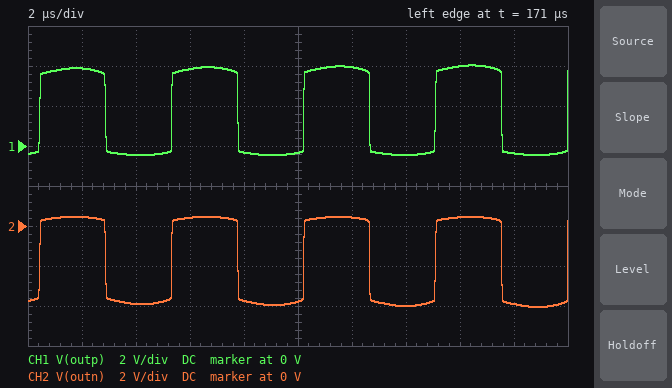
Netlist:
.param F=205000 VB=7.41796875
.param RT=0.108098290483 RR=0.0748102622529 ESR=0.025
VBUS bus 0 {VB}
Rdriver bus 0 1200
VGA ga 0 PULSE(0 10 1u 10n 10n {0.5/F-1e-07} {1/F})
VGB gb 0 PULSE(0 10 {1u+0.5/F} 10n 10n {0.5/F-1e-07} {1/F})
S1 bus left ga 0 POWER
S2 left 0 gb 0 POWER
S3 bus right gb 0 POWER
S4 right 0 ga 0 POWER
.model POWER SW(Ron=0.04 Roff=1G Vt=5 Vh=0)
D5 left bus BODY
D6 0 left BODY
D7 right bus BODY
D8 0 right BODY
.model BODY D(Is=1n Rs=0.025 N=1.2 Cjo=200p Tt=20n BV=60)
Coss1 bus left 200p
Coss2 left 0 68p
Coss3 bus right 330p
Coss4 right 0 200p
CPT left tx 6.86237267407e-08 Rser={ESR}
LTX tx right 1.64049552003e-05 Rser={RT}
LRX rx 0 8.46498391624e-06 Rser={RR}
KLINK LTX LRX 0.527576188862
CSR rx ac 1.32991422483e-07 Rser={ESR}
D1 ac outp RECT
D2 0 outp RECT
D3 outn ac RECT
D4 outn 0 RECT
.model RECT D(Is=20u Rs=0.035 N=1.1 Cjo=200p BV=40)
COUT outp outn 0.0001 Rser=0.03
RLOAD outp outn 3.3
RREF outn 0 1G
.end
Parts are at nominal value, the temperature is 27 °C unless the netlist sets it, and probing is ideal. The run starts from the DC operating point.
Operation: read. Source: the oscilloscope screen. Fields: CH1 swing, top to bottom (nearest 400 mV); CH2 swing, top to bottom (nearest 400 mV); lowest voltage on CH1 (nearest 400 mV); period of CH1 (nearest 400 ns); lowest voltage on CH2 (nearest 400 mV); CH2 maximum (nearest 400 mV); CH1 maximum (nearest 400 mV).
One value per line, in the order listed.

4.4 V
4.4 V
-400 mV
4.8 µs
-4.0 V
400 mV
4.0 V
